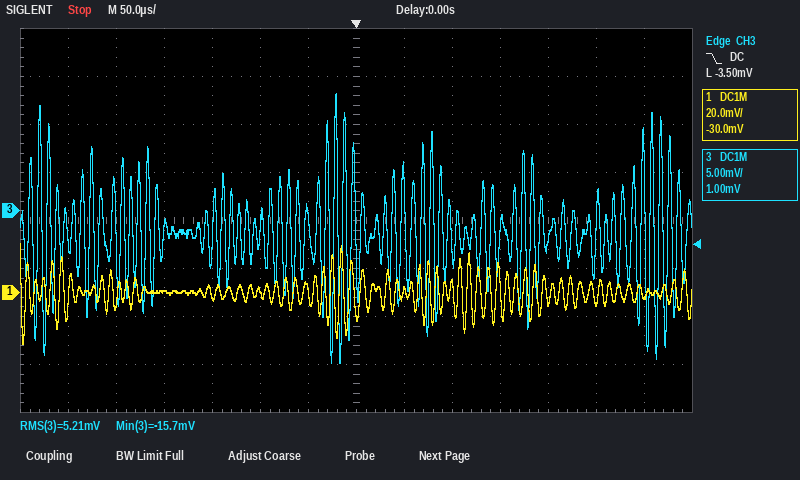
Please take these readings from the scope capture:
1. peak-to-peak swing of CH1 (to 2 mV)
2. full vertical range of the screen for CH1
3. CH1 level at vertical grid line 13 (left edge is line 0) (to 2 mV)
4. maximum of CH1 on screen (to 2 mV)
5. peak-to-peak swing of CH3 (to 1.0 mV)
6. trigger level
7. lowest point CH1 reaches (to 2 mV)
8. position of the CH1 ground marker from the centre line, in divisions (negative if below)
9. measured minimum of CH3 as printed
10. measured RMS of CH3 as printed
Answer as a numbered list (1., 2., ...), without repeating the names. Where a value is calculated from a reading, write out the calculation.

1. 20 mV − (-22 mV) = 42 mV
2. 160 mV
3. -2 mV
4. 20 mV
5. 28.0 mV
6. -3.50 mV
7. -22 mV
8. -1.5 div
9. -15.7 mV
10. 5.21 mV
